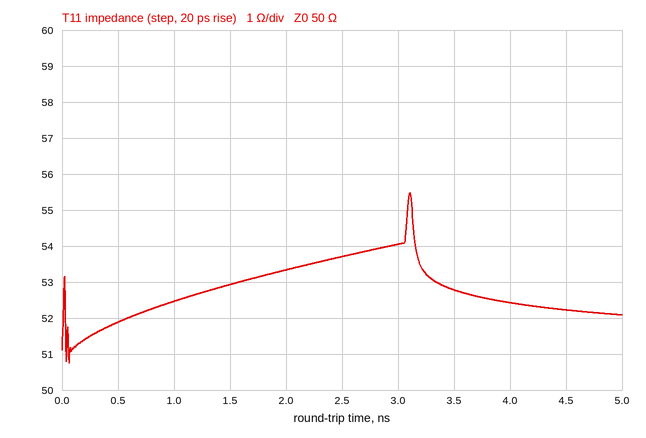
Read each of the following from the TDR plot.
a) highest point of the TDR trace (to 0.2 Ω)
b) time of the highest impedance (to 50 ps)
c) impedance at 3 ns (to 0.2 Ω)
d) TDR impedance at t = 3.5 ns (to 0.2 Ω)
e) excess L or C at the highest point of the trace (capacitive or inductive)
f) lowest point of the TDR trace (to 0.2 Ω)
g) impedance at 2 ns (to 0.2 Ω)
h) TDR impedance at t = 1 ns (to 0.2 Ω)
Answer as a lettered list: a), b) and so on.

a) 55.4 Ω
b) 3.10 ns
c) 54.0 Ω
d) 52.8 Ω
e) inductive
f) 50.8 Ω
g) 53.4 Ω
h) 52.4 Ω
